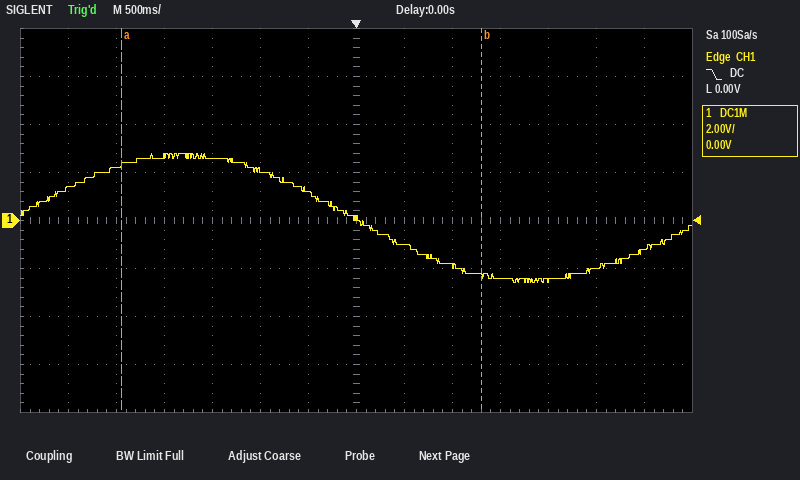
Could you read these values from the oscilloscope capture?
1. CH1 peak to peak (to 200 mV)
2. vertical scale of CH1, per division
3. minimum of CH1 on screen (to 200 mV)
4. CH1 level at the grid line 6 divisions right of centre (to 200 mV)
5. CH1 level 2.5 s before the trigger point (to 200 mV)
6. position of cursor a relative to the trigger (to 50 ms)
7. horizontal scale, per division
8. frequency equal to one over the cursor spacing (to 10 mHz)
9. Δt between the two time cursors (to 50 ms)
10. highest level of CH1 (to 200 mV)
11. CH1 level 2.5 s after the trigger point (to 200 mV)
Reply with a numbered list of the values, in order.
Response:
1. 5.4 V
2. 2 V
3. -2.6 V
4. -1.2 V
5. 2.2 V
6. -2.45 s
7. 500 ms
8. 270 mHz
9. 3.75 s
10. 2.8 V
11. -2.0 V
